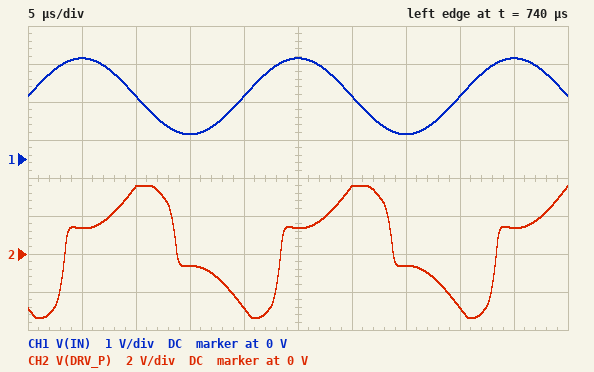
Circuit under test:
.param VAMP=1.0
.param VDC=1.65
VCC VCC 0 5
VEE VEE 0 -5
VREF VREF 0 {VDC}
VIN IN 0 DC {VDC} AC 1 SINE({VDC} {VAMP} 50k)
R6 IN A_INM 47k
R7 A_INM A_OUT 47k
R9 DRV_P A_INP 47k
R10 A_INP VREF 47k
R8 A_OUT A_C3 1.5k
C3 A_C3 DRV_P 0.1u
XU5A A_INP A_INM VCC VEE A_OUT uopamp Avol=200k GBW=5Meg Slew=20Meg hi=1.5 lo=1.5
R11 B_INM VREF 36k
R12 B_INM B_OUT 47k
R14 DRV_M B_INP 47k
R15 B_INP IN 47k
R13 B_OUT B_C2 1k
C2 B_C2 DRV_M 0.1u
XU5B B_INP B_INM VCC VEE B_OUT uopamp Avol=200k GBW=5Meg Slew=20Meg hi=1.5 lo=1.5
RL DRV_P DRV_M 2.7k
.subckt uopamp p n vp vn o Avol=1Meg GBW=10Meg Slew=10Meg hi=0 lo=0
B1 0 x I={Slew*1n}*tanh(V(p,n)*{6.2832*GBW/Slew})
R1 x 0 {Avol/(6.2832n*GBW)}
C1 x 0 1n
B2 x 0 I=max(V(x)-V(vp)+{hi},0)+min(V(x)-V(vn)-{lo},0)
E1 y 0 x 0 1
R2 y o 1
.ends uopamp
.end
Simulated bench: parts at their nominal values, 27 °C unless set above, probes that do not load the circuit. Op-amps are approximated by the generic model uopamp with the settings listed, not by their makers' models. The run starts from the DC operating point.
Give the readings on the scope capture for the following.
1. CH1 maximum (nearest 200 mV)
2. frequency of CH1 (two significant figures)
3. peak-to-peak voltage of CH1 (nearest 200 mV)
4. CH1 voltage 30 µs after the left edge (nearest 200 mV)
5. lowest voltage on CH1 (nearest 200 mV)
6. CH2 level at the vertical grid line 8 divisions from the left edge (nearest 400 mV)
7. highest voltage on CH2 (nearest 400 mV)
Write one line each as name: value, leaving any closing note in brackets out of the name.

CH1 maximum: 2.6 V
frequency of CH1: 50 kHz
peak-to-peak voltage of CH1: 2.0 V
CH1 voltage 30 µs after the left edge: 1.6 V
lowest voltage on CH1: 600 mV
CH2 level at the vertical grid line 8 divisions from the left edge: -2.8 V
highest voltage on CH2: 3.6 V
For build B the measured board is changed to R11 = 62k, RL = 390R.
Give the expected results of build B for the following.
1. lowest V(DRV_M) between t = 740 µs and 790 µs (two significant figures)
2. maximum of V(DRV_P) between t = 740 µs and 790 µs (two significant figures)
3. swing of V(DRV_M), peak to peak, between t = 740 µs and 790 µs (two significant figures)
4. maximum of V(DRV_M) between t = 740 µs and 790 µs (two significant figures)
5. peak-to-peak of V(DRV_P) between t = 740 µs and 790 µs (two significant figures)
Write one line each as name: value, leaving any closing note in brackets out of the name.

lowest V(DRV_M) between t = 740 µs and 790 µs: 140 mV
maximum of V(DRV_P) between t = 740 µs and 790 µs: 2.7 V
swing of V(DRV_M), peak to peak, between t = 740 µs and 790 µs: 2.8 V
maximum of V(DRV_M) between t = 740 µs and 790 µs: 2.9 V
peak-to-peak of V(DRV_P) between t = 740 µs and 790 µs: 2.3 V
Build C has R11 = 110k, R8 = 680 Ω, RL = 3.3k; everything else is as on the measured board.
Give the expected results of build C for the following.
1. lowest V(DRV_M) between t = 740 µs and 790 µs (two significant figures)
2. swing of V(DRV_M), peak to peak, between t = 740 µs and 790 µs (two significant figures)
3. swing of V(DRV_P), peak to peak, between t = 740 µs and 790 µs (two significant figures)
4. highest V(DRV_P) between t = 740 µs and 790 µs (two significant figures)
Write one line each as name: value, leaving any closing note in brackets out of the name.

lowest V(DRV_M) between t = 740 µs and 790 µs: 280 mV
swing of V(DRV_M), peak to peak, between t = 740 µs and 790 µs: 2.1 V
swing of V(DRV_P), peak to peak, between t = 740 µs and 790 µs: 6.1 V
highest V(DRV_P) between t = 740 µs and 790 µs: 3.4 V
